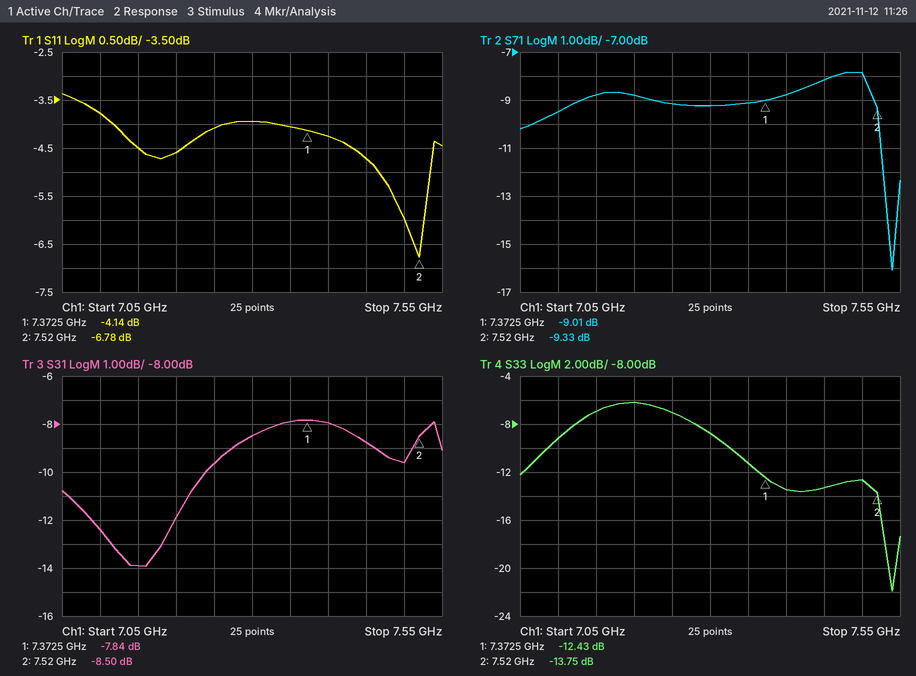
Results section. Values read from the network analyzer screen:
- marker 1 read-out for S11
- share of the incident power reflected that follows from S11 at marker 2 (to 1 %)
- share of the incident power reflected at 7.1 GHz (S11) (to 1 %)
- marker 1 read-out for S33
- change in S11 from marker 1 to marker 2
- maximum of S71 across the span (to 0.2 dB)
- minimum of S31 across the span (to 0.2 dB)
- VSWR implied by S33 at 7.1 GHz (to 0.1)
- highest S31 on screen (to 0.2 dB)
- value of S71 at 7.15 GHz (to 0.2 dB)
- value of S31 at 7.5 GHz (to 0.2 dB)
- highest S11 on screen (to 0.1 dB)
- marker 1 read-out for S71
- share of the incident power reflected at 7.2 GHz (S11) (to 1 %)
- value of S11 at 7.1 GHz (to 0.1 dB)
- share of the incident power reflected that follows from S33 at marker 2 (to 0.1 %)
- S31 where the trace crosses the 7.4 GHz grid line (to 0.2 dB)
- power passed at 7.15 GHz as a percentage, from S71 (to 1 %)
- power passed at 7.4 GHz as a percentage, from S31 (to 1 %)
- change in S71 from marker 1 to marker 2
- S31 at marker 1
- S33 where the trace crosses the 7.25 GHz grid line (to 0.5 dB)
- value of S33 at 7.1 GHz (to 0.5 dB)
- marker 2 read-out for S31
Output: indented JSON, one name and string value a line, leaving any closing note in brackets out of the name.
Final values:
{
  "marker 1 read-out for S11": "-4.14 dB",
  "share of the incident power reflected that follows from S11 at marker 2": "21 %",
  "share of the incident power reflected at 7.1 GHz (S11)": "42 %",
  "marker 1 read-out for S33": "-12.43 dB",
  "change in S11 from marker 1 to marker 2": "-2.64 dB",
  "maximum of S71 across the span": "-7.8 dB",
  "minimum of S31 across the span": "-14.0 dB",
  "VSWR implied by S33 at 7.1 GHz": "2.1",
  "highest S31 on screen": "-7.8 dB",
  "value of S71 at 7.15 GHz": "-8.8 dB",
  "value of S31 at 7.5 GHz": "-9.6 dB",
  "highest S11 on screen": "-3.4 dB",
  "marker 1 read-out for S71": "-9.01 dB",
  "share of the incident power reflected at 7.2 GHz (S11)": "35 %",
  "value of S11 at 7.1 GHz": "-3.8 dB",
  "share of the incident power reflected that follows from S33 at marker 2": "4.2 %",
  "S31 where the trace crosses the 7.4 GHz grid line": "-8.0 dB",
  "power passed at 7.15 GHz as a percentage, from S71": "13 %",
  "power passed at 7.4 GHz as a percentage, from S31": "16 %",
  "change in S71 from marker 1 to marker 2": "-0.32 dB",
  "S31 at marker 1": "-7.84 dB",
  "S33 where the trace crosses the 7.25 GHz grid line": "-7.0 dB",
  "value of S33 at 7.1 GHz": "-9.0 dB",
  "marker 2 read-out for S31": "-8.50 dB"
}
